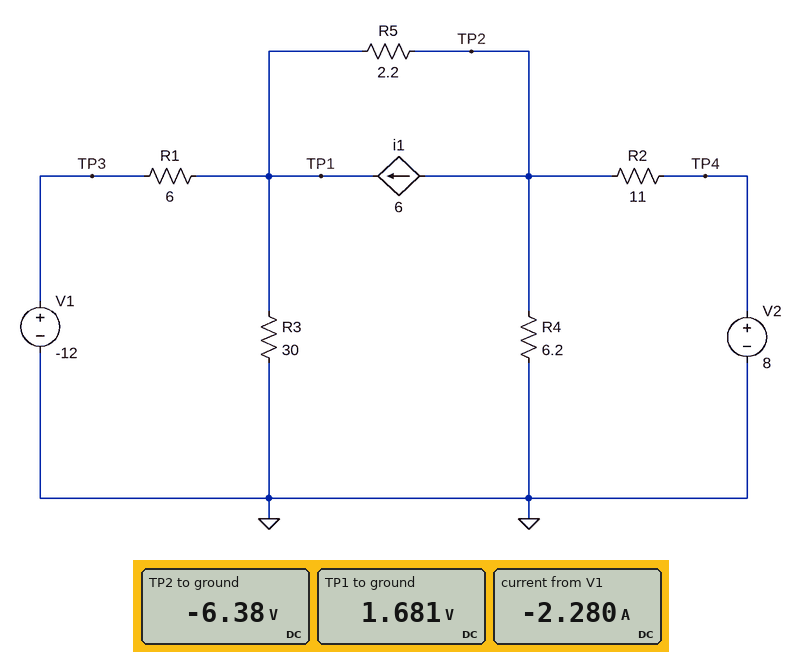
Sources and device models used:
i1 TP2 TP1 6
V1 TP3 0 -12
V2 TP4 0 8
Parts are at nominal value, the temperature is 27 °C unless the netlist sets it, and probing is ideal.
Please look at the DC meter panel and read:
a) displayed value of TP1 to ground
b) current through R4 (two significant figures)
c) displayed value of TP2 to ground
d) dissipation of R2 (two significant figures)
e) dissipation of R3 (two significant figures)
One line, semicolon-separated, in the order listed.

1.681 V; 1.0 A; -6.38 V; 19 W; 94 mW
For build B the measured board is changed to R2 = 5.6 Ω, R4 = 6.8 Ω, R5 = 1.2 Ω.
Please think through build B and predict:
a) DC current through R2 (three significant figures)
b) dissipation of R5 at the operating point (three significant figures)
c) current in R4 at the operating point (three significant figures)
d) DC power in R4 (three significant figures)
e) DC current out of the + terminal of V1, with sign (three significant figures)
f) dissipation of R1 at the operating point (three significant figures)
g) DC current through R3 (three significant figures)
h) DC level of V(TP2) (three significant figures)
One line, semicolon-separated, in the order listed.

1.92 A; 16.2 W; 406 mA; 1.12 W; -2.27 A; 31.0 W; 54.7 mA; -2.76 V
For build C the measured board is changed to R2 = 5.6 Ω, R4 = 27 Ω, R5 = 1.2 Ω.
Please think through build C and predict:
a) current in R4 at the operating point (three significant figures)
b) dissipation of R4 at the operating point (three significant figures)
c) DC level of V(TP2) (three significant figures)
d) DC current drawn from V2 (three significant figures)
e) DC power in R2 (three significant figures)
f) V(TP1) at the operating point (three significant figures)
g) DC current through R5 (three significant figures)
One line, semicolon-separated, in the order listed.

132 mA; 472 mW; -3.57 V; 2.07 A; 23.9 W; 992 mV; 3.80 A
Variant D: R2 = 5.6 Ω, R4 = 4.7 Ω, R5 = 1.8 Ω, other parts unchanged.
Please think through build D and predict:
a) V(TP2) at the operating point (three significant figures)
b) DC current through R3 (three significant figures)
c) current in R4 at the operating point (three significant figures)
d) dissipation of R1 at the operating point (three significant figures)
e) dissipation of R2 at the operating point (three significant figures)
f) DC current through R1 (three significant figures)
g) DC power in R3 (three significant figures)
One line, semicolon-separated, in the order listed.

-3.03 V; 102 mA; 644 mA; 37.8 W; 21.7 W; 2.51 A; 314 mW
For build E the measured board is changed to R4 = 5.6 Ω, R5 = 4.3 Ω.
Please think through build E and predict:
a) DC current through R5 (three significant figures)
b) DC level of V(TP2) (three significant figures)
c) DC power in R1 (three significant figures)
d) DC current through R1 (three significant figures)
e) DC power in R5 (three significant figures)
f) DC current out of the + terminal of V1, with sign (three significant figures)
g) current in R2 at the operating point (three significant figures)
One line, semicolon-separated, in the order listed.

3.04 A; -8.28 V; 47.0 W; 2.80 A; 39.8 W; -2.80 A; 1.48 A
